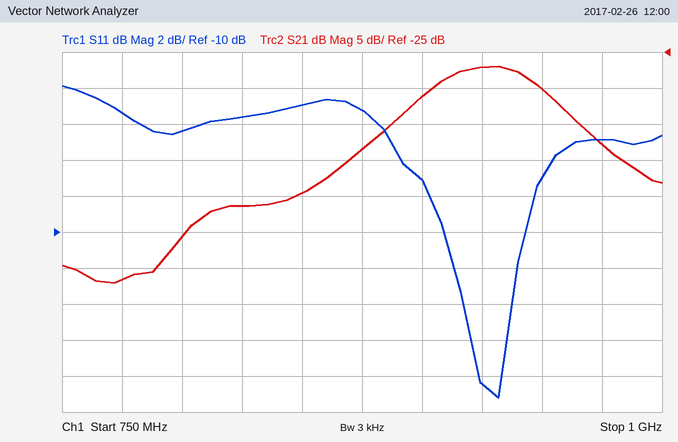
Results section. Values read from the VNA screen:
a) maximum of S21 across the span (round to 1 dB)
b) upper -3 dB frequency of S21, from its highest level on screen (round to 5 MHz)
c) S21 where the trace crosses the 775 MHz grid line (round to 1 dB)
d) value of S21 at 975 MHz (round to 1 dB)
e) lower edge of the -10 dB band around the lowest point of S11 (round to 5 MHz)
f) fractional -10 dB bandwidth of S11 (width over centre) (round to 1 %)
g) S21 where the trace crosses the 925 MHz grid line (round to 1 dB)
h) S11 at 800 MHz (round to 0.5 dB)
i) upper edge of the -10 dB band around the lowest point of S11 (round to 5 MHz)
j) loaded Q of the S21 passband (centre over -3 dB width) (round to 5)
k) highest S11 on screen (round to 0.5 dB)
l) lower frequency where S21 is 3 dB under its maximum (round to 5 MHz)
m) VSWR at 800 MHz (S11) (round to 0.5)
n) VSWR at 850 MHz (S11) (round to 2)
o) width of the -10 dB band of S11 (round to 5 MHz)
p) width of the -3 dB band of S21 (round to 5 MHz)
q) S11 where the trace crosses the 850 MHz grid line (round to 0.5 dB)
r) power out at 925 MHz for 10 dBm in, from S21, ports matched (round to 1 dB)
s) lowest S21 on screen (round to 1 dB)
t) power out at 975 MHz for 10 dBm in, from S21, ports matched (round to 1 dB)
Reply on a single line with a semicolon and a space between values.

-27 dB; 950 MHz; -57 dB; -38 dB; 910 MHz; 4 %; -27 dB; -4.5 dB; 945 MHz; 20; -2.0 dB; 905 MHz; 4.0; 6; 35 MHz; 45 MHz; -3.0 dB; -17 dBm; -57 dB; -28 dBm
